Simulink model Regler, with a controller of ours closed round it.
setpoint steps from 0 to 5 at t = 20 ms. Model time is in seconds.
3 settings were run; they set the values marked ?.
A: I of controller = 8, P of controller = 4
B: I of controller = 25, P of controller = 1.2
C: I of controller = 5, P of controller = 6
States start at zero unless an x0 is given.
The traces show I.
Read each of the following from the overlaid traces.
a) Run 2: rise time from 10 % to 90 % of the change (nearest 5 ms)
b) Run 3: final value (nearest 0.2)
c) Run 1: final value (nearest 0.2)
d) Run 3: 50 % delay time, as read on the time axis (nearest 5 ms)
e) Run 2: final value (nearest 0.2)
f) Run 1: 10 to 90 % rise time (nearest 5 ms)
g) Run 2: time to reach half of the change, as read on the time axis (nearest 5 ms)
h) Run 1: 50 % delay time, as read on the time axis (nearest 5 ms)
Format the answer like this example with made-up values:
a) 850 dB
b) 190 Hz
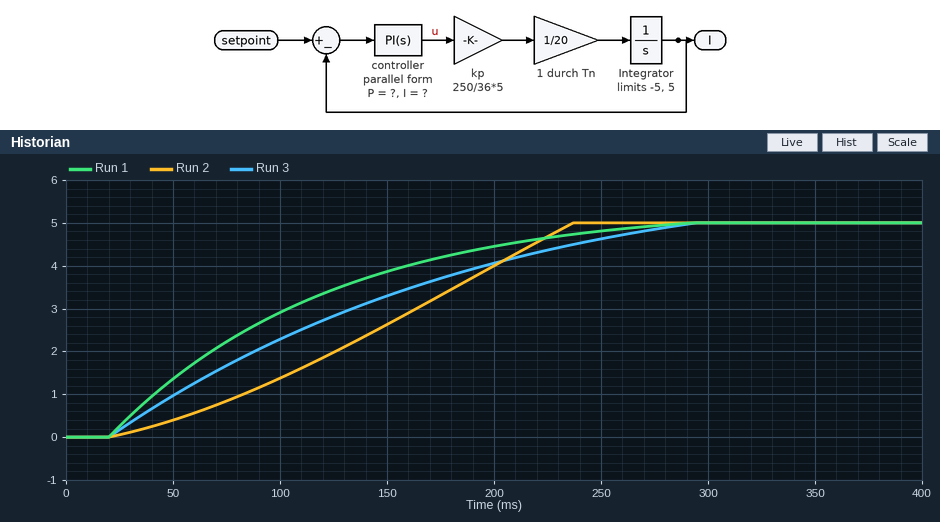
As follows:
a) 160 ms
b) 5.0
c) 5.0
d) 110 ms
e) 5.0
f) 175 ms
g) 145 ms
h) 85 ms
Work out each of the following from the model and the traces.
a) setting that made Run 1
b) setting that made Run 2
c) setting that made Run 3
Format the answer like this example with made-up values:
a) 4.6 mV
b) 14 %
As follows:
a) C
b) B
c) A
